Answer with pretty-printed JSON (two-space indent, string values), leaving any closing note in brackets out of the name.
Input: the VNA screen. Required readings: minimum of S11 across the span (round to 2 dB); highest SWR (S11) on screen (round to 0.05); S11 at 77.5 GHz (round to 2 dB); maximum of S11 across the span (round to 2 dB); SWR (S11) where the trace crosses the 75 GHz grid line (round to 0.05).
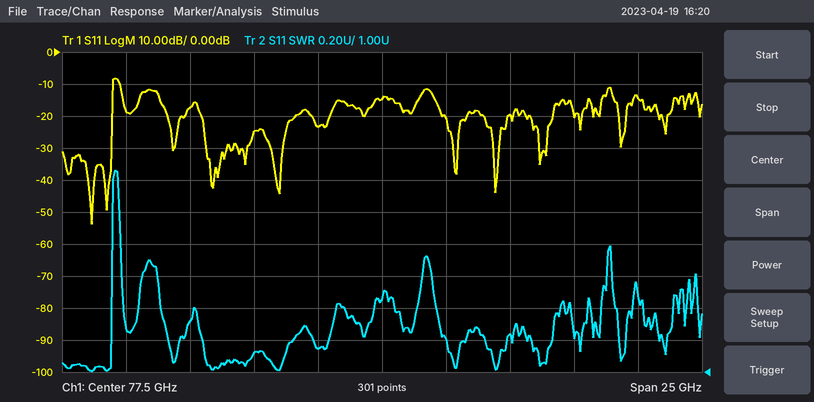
{
  "minimum of S11 across the span": "-54 dB",
  "highest SWR (S11) on screen": "2.25",
  "S11 at 77.5 GHz": "-14 dB",
  "maximum of S11 across the span": "-8 dB",
  "SWR (S11) where the trace crosses the 75 GHz grid line": "1.15"
}
